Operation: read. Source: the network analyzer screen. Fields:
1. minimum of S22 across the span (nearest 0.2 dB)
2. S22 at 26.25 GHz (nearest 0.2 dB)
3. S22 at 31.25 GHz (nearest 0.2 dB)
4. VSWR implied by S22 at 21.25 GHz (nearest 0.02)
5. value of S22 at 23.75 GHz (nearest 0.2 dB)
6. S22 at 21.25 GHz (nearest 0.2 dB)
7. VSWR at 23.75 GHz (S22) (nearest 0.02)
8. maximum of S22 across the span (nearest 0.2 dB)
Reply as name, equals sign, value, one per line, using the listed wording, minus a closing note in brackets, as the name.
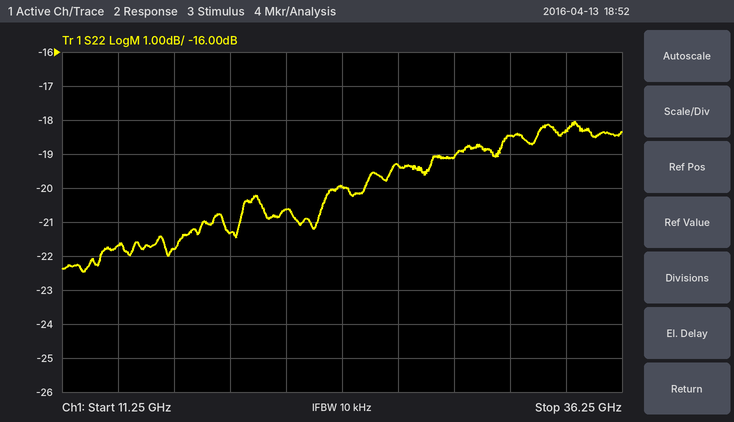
minimum of S22 across the span = -22.4 dB
S22 at 26.25 GHz = -19.4 dB
S22 at 31.25 GHz = -18.4 dB
VSWR implied by S22 at 21.25 GHz = 1.20
value of S22 at 23.75 GHz = -20.0 dB
S22 at 21.25 GHz = -20.6 dB
VSWR at 23.75 GHz (S22) = 1.22
maximum of S22 across the span = -18.0 dB
